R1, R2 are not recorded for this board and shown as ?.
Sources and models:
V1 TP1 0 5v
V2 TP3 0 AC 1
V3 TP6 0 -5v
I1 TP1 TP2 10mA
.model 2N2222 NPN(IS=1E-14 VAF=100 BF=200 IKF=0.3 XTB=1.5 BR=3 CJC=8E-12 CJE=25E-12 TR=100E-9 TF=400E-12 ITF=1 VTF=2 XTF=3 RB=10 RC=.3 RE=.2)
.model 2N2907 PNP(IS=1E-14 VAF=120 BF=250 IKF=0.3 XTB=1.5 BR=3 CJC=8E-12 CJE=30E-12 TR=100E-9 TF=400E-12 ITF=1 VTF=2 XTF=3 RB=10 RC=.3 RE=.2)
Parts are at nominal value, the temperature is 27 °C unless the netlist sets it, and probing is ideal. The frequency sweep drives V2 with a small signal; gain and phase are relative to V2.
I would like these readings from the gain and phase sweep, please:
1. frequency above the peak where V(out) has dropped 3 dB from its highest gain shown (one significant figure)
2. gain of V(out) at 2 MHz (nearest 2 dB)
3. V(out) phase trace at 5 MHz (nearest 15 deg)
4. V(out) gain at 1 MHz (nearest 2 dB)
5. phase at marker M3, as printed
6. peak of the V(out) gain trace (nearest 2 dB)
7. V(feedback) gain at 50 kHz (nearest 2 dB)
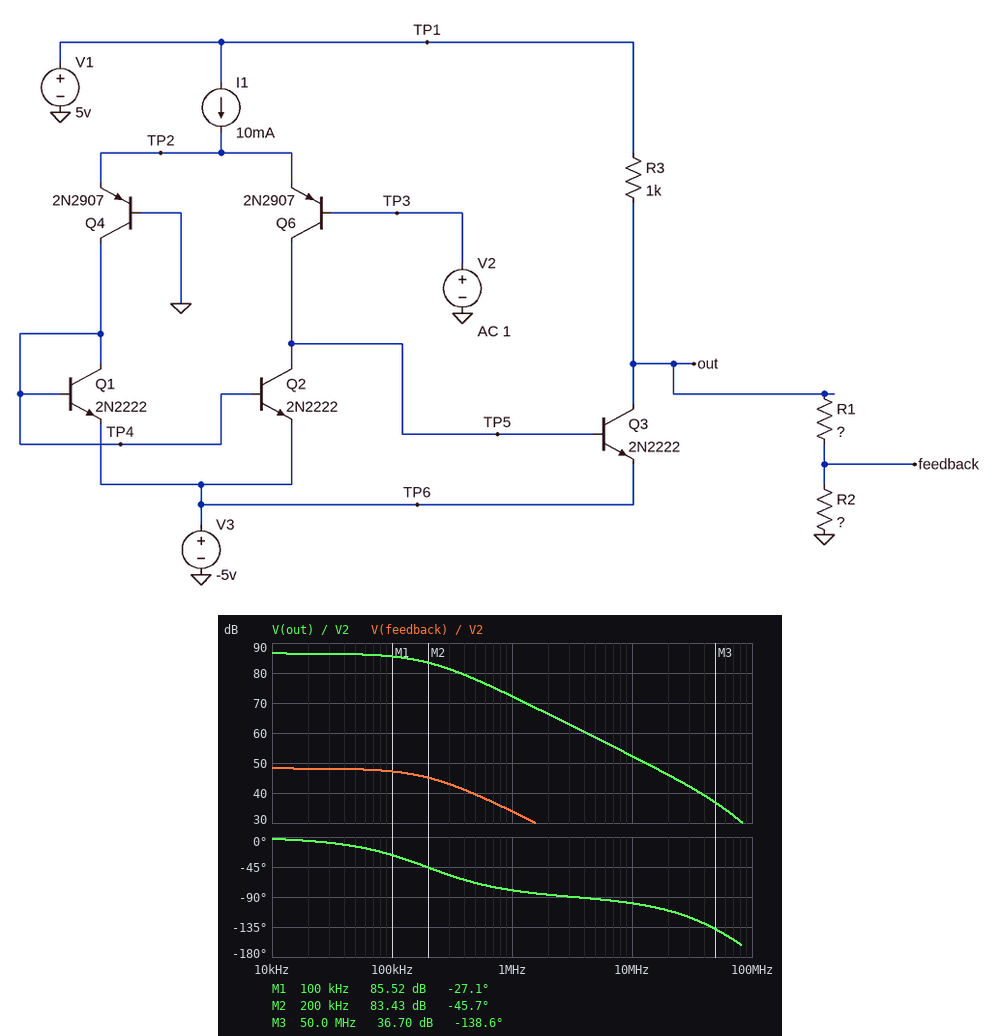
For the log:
200 kHz
66 dB
-90 deg
72 dB
-138.6 deg
86 dB
48 dB
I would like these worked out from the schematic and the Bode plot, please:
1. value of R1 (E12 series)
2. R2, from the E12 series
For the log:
2.2 kΩ
27 Ω
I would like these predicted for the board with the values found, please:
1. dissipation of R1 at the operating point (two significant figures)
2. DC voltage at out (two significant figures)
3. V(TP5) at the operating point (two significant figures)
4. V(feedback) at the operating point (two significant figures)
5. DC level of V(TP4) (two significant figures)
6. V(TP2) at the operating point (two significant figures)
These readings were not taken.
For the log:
4.3 mW
-3.1 V
-4.3 V
-38 mV
-4.3 V
700 mV
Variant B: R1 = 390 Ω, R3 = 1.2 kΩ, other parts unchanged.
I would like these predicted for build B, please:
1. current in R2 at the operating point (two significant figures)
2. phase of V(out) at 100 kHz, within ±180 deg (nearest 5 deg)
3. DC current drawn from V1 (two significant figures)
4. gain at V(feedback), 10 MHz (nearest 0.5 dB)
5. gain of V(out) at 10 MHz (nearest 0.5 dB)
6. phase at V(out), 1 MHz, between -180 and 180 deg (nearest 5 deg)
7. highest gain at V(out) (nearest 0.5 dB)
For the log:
4.1 mA
-15 deg
16 mA
28.5 dB
52.0 dB
-70 deg
80.0 dB
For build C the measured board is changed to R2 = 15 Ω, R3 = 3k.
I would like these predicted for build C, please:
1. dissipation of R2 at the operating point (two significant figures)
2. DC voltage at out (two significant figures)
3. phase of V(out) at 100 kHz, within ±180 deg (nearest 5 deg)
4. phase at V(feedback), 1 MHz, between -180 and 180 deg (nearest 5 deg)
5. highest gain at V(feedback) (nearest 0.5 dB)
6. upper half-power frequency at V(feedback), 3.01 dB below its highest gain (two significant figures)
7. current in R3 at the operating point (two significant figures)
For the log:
73 µW
-4.9 V
-10 deg
-65 deg
3.0 dB
510 kHz
3.3 mA
